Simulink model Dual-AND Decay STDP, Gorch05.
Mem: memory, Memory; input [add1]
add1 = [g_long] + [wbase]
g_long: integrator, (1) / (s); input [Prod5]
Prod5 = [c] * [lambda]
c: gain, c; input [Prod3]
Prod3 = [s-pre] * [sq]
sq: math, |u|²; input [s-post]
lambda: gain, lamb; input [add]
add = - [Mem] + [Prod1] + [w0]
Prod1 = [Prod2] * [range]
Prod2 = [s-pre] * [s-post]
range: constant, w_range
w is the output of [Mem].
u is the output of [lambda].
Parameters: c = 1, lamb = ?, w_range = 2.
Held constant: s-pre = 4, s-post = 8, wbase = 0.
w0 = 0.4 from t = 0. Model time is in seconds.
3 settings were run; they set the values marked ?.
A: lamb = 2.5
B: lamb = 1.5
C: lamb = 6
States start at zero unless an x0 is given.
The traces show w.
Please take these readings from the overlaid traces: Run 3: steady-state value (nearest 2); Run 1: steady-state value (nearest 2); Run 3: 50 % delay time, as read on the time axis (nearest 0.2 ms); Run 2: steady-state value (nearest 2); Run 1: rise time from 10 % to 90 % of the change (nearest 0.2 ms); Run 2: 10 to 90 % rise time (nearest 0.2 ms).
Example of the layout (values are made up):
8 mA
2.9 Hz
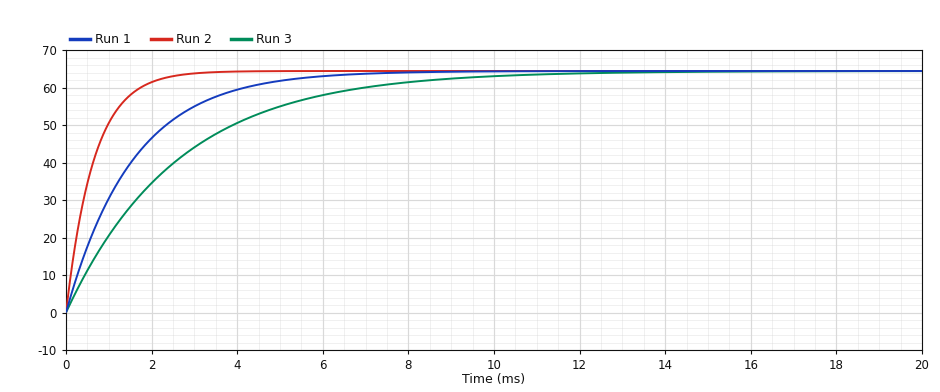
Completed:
64
64
1.8 ms
64
3.4 ms
1.4 ms
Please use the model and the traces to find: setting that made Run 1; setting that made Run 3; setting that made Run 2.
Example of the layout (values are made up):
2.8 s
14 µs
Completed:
A
B
C
